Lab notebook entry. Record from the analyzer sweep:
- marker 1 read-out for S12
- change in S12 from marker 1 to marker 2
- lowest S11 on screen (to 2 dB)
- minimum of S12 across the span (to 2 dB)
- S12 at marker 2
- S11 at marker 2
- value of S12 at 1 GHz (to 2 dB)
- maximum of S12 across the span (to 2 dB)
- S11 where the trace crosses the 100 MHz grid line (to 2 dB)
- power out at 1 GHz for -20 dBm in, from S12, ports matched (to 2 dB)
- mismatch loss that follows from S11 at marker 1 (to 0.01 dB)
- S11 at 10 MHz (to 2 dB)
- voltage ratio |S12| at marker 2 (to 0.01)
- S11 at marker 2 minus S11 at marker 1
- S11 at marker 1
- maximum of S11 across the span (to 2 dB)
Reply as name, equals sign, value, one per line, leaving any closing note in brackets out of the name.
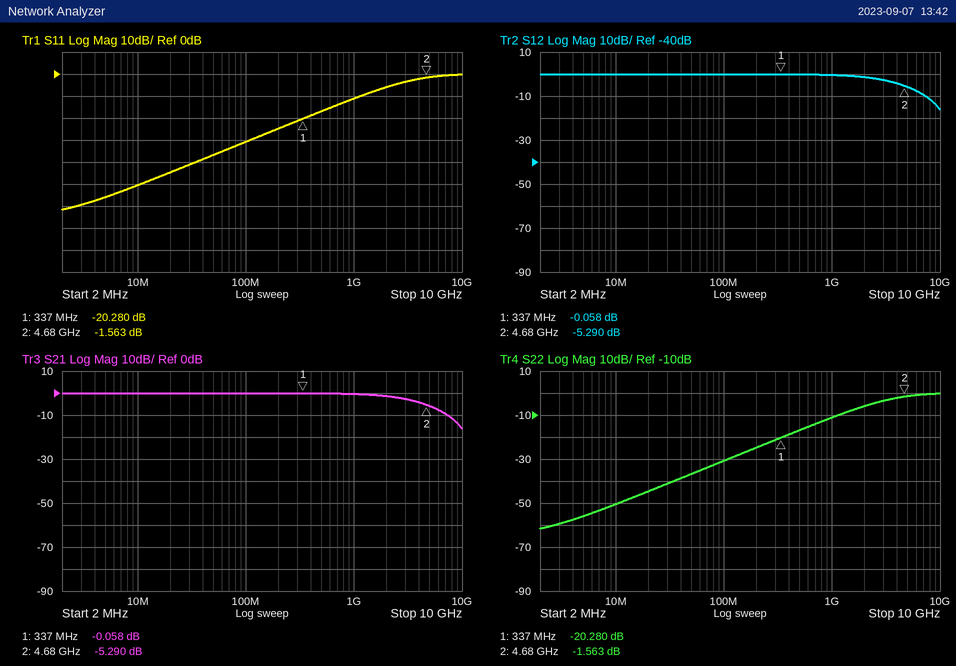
marker 1 read-out for S12 = -0.058 dB
change in S12 from marker 1 to marker 2 = -5.232 dB
lowest S11 on screen = -62 dB
minimum of S12 across the span = -16 dB
S12 at marker 2 = -5.290 dB
S11 at marker 2 = -1.563 dB
value of S12 at 1 GHz = 0 dB
maximum of S12 across the span = 0 dB
S11 where the trace crosses the 100 MHz grid line = -30 dB
power out at 1 GHz for -20 dBm in, from S12, ports matched = -20 dBm
mismatch loss that follows from S11 at marker 1 = 0.04 dB
S11 at 10 MHz = -50 dB
voltage ratio |S12| at marker 2 = 0.54
S11 at marker 2 minus S11 at marker 1 = 18.717 dB
S11 at marker 1 = -20.280 dB
maximum of S11 across the span = 0 dB
